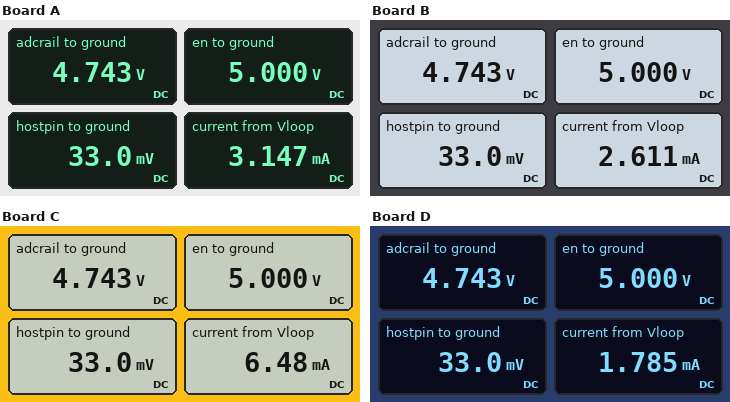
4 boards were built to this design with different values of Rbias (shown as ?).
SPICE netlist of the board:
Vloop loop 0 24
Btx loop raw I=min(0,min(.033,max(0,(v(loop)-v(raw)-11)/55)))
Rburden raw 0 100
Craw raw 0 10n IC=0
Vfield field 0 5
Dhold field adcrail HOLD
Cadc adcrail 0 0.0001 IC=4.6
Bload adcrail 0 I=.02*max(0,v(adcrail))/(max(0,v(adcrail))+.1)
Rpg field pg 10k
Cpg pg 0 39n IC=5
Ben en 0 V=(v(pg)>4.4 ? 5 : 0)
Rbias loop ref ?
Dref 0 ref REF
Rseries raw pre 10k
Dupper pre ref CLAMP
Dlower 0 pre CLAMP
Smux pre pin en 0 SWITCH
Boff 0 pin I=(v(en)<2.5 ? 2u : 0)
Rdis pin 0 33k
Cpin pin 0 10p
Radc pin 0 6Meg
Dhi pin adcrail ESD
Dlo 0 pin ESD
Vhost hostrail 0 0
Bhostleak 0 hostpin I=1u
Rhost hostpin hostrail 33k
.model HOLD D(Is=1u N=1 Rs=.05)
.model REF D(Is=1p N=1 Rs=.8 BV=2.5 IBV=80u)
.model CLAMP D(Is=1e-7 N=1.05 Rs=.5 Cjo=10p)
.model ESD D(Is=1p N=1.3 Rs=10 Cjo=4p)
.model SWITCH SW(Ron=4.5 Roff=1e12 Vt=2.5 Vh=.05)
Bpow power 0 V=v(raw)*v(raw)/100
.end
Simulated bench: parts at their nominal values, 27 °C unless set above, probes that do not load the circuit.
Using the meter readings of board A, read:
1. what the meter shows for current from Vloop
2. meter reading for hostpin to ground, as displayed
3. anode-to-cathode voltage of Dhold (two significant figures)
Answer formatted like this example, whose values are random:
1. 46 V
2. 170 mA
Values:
1. 3.147 mA
2. 33.0 mV
3. 260 mV
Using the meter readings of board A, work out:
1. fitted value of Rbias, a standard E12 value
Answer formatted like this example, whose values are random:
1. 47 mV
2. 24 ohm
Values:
1. 6.8 kΩ
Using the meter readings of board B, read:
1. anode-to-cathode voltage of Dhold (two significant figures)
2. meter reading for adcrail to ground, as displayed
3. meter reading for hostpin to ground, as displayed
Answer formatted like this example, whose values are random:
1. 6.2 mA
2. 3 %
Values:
1. 260 mV
2. 4.743 V
3. 33.0 mV
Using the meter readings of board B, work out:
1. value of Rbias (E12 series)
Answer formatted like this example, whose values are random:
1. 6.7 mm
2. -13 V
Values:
1. 8.2 kΩ
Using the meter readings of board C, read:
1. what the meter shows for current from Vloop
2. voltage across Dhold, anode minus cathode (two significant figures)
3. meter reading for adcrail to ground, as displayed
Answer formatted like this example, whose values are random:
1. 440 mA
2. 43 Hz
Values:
1. 6.48 mA
2. 260 mV
3. 4.743 V
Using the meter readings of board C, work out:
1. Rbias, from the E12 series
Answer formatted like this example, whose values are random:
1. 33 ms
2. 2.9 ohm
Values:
1. 3.3 kΩ
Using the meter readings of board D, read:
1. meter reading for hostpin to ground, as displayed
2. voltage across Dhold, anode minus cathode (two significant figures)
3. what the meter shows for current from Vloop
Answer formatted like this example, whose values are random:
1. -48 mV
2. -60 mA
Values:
1. 33.0 mV
2. 260 mV
3. 1.785 mA
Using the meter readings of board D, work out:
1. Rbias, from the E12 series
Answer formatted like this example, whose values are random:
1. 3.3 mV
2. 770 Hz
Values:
1. 12 kΩ
